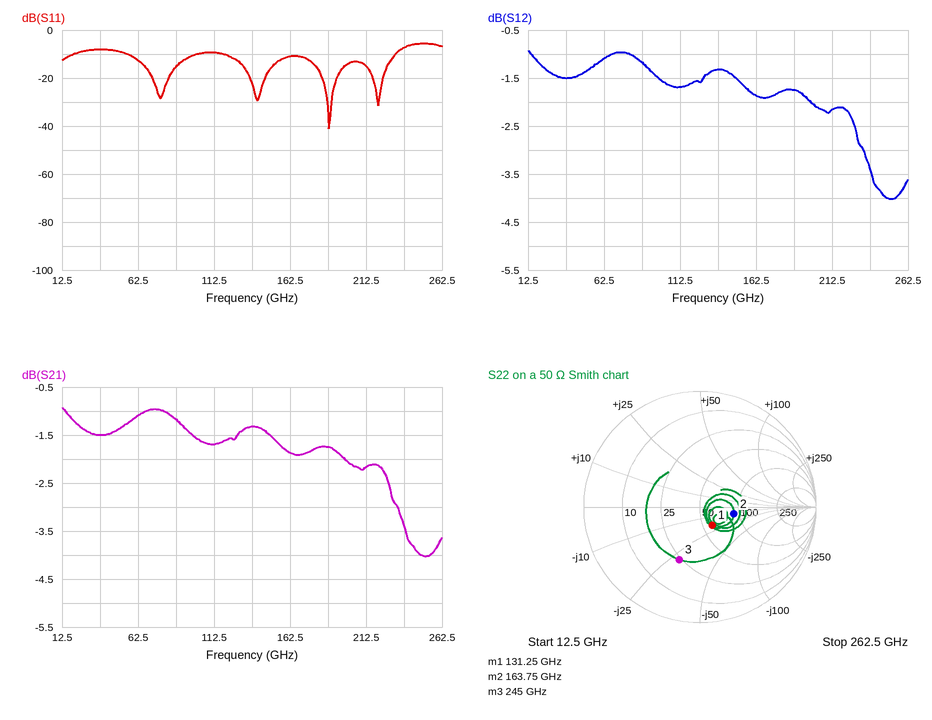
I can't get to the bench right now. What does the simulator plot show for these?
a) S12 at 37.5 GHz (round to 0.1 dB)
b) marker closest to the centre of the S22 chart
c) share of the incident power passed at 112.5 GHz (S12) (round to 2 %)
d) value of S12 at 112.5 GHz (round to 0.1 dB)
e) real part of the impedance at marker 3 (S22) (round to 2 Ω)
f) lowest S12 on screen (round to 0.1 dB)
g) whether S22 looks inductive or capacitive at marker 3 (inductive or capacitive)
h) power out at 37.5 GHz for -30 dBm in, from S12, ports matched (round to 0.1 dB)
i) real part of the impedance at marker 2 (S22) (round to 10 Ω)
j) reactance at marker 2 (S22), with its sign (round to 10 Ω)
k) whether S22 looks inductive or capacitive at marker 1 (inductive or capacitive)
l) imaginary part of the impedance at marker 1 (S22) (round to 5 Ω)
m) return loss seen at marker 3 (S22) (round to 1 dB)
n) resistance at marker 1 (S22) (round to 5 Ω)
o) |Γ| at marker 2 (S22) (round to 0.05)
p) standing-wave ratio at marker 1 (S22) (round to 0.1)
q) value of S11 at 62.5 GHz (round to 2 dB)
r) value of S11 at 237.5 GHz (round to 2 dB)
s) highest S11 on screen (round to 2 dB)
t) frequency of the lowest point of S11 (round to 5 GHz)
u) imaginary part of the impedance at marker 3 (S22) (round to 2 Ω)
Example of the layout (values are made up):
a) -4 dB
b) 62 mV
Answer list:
a) -1.5 dB
b) marker 1
c) 68 %
d) -1.7 dB
e) 24 Ω
f) -4.0 dB
g) capacitive
h) -31.5 dBm
i) 90 Ω
j) -10 Ω
k) capacitive
l) -20 Ω
m) 6 dB
n) 60 Ω
o) 0.30
p) 1.5
q) -12 dB
r) -8 dB
s) -6 dB
t) 190 GHz
u) -28 Ω
